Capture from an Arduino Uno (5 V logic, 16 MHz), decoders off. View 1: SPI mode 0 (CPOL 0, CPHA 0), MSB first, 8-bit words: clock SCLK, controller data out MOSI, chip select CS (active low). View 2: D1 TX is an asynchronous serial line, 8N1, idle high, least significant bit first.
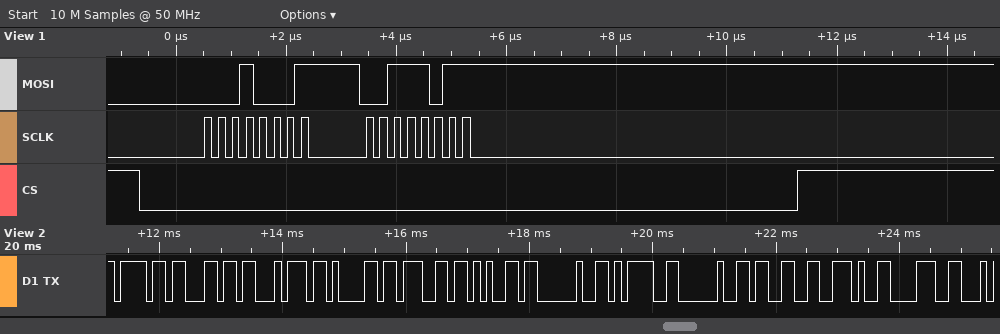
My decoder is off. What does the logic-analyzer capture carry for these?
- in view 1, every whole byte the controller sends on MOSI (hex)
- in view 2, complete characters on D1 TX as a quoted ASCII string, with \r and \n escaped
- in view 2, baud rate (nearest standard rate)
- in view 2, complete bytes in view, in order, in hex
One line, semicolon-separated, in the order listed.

11 3B; "oltage = 3.8"; 9600 baud; 6F 6C 74 61 67 65 20 3D 20 33 2E 38
